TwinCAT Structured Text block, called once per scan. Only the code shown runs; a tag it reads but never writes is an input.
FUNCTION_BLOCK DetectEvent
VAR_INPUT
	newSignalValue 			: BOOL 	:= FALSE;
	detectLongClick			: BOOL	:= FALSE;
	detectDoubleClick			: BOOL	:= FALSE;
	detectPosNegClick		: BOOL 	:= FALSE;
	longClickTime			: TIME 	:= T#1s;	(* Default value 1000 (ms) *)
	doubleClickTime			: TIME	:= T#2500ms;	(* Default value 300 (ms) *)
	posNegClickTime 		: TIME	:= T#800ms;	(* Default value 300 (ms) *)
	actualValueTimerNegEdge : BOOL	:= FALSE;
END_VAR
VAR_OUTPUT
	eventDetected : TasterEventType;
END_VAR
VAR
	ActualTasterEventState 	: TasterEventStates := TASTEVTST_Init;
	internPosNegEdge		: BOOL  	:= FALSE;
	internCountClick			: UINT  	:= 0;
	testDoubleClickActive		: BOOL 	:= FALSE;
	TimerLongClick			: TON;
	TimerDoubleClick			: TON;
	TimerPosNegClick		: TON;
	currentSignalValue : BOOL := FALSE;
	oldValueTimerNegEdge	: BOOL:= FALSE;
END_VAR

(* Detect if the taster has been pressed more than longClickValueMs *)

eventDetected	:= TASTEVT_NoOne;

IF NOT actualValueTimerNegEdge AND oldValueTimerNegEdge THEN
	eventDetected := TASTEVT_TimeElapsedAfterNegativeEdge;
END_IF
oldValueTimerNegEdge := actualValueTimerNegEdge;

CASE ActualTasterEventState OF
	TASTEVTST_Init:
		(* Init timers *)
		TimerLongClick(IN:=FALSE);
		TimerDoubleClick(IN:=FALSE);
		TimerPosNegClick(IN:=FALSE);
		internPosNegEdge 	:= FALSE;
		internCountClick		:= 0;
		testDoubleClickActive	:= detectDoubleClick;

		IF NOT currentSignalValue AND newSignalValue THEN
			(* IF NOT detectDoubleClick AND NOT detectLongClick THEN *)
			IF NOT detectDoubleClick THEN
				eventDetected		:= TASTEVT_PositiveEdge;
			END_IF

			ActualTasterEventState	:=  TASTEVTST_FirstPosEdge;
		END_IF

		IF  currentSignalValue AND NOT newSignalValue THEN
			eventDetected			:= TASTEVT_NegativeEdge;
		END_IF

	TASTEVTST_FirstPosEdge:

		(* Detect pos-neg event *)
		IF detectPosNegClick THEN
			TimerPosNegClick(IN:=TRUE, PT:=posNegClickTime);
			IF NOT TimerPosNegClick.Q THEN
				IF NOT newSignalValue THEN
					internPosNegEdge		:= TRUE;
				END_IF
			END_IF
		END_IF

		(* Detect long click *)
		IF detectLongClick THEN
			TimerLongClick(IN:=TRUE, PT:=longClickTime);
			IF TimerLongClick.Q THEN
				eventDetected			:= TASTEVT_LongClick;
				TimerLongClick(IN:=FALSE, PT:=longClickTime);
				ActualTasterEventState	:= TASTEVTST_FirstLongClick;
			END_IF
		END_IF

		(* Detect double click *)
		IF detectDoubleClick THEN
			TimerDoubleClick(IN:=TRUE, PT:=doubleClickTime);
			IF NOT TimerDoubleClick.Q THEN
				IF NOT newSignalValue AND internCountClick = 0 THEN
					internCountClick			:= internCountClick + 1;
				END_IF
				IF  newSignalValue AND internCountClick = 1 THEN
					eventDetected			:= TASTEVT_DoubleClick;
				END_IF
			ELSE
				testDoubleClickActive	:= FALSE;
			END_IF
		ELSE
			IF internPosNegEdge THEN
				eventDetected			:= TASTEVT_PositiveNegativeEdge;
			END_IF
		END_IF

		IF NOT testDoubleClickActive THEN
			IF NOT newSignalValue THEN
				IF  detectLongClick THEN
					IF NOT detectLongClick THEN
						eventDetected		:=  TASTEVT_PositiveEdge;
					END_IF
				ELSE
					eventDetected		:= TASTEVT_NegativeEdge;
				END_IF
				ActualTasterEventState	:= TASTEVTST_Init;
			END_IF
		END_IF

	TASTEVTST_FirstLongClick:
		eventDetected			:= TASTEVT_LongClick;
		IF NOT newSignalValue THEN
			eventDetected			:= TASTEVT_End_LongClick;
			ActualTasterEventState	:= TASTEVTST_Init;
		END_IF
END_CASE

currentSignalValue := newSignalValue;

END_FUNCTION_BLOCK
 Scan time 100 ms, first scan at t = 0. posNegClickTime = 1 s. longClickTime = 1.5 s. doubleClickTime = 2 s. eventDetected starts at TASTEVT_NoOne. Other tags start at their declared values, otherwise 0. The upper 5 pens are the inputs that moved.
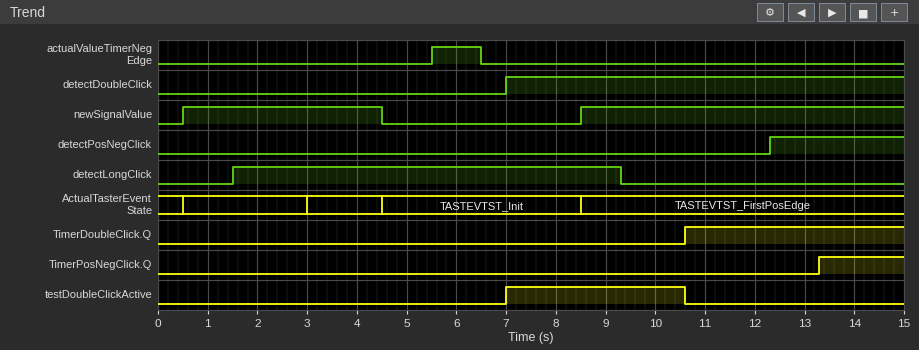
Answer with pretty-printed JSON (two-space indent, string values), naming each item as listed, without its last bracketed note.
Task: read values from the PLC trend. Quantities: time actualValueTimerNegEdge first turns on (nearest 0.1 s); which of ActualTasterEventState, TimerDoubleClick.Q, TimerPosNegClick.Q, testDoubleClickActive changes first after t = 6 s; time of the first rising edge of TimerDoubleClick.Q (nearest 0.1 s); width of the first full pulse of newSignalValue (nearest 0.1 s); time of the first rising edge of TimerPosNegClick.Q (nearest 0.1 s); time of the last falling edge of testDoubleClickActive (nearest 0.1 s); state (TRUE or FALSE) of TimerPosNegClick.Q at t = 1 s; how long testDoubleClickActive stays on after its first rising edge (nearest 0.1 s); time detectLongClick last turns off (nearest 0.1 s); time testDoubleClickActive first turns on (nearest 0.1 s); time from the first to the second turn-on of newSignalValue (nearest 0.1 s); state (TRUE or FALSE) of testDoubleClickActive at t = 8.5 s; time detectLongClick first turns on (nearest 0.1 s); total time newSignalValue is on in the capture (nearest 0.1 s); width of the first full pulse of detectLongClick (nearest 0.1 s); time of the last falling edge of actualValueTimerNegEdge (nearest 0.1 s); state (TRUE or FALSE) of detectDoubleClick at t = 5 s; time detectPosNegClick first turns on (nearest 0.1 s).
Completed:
{
  "time actualValueTimerNegEdge first turns on": "5.5 s",
  "which of ActualTasterEventState, TimerDoubleClick.Q, TimerPosNegClick.Q, testDoubleClickActive changes first after t = 6 s": "testDoubleClickActive",
  "time of the first rising edge of TimerDoubleClick.Q": "10.6 s",
  "width of the first full pulse of newSignalValue": "4.0 s",
  "time of the first rising edge of TimerPosNegClick.Q": "13.3 s",
  "time of the last falling edge of testDoubleClickActive": "10.6 s",
  "state (TRUE or FALSE) of TimerPosNegClick.Q at t = 1 s": "FALSE",
  "how long testDoubleClickActive stays on after its first rising edge": "3.6 s",
  "time detectLongClick last turns off": "9.3 s",
  "time testDoubleClickActive first turns on": "7.0 s",
  "time from the first to the second turn-on of newSignalValue": "8.0 s",
  "state (TRUE or FALSE) of testDoubleClickActive at t = 8.5 s": "TRUE",
  "time detectLongClick first turns on": "1.5 s",
  "total time newSignalValue is on in the capture": "10.5 s",
  "width of the first full pulse of detectLongClick": "7.8 s",
  "time of the last falling edge of actualValueTimerNegEdge": "6.5 s",
  "state (TRUE or FALSE) of detectDoubleClick at t = 5 s": "FALSE",
  "time detectPosNegClick first turns on": "12.3 s"
}
